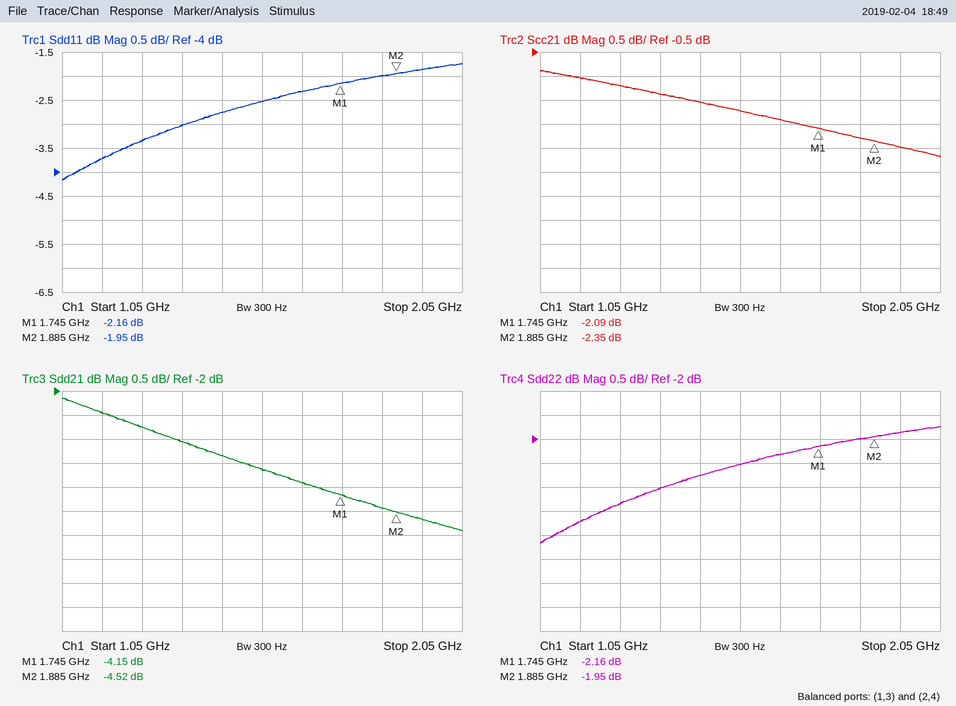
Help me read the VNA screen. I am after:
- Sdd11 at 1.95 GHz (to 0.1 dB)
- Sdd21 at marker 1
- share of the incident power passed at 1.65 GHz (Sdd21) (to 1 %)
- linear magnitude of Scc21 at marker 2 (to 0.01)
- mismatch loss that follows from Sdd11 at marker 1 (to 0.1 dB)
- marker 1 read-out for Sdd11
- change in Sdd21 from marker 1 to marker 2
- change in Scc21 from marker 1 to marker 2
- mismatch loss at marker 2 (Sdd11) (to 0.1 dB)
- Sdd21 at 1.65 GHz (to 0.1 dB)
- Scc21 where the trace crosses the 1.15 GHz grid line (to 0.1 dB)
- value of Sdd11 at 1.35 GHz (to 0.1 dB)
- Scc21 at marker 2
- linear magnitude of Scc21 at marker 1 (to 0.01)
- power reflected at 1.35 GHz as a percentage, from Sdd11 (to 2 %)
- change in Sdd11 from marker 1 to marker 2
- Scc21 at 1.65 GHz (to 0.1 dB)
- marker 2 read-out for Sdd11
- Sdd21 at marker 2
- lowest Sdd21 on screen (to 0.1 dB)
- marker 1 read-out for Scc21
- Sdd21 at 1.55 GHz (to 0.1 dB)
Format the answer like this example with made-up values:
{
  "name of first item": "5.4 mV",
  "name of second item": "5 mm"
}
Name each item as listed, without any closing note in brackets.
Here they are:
{
  "Sdd11 at 1.95 GHz": "-1.9 dB",
  "Sdd21 at marker 1": "-4.15 dB",
  "share of the incident power passed at 1.65 GHz (Sdd21)": "41 %",
  "linear magnitude of Scc21 at marker 2": "0.76",
  "mismatch loss that follows from Sdd11 at marker 1": "4.1 dB",
  "marker 1 read-out for Sdd11": "-2.16 dB",
  "change in Sdd21 from marker 1 to marker 2": "-0.37 dB",
  "change in Scc21 from marker 1 to marker 2": "-0.26 dB",
  "mismatch loss at marker 2 (Sdd11)": "4.4 dB",
  "Sdd21 at 1.65 GHz": "-3.9 dB",
  "Scc21 where the trace crosses the 1.15 GHz grid line": "-1.0 dB",
  "value of Sdd11 at 1.35 GHz": "-3.0 dB",
  "Scc21 at marker 2": "-2.35 dB",
  "linear magnitude of Scc21 at marker 1": "0.79",
  "power reflected at 1.35 GHz as a percentage, from Sdd11": "50 %",
  "change in Sdd11 from marker 1 to marker 2": "0.21 dB",
  "Scc21 at 1.65 GHz": "-1.9 dB",
  "marker 2 read-out for Sdd11": "-1.95 dB",
  "Sdd21 at marker 2": "-4.52 dB",
  "lowest Sdd21 on screen": "-4.9 dB",
  "marker 1 read-out for Scc21": "-2.09 dB",
  "Sdd21 at 1.55 GHz": "-3.6 dB"
}
